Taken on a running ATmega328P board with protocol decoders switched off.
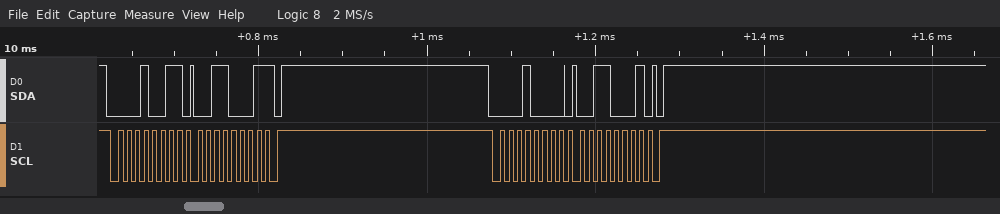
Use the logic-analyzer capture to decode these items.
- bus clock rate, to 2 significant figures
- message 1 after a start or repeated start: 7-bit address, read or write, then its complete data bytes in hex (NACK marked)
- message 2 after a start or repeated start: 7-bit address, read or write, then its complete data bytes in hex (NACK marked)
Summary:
100 kHz
0x09 read: 31 NACK
0x08 write: 31
